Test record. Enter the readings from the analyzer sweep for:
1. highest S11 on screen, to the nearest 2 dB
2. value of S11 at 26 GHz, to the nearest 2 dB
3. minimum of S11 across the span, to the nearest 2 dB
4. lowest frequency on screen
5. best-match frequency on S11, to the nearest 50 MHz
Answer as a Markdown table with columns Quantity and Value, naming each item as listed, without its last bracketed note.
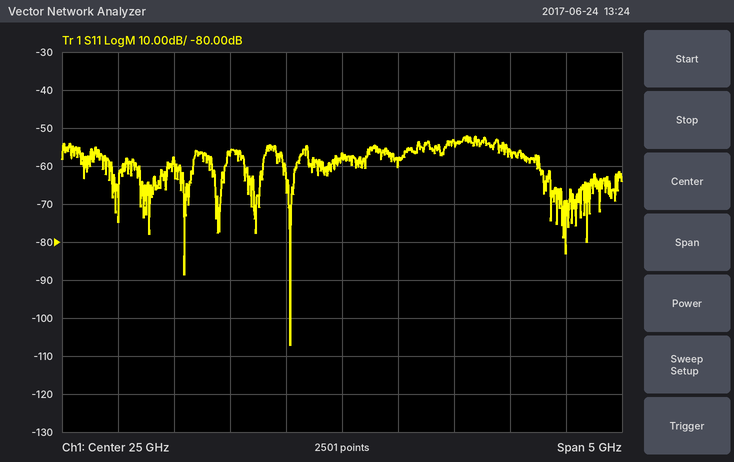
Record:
| Quantity | Value |
|---|---|
| highest S11 on screen, to the nearest 2 dB | -52 dB |
| value of S11 at 26 GHz, to the nearest 2 dB | -54 dB |
| minimum of S11 across the span, to the nearest 2 dB | -108 dB |
| lowest frequency on screen | 22.5 GHz |
| best-match frequency on S11, to the nearest 50 MHz | 24.55 GHz |
